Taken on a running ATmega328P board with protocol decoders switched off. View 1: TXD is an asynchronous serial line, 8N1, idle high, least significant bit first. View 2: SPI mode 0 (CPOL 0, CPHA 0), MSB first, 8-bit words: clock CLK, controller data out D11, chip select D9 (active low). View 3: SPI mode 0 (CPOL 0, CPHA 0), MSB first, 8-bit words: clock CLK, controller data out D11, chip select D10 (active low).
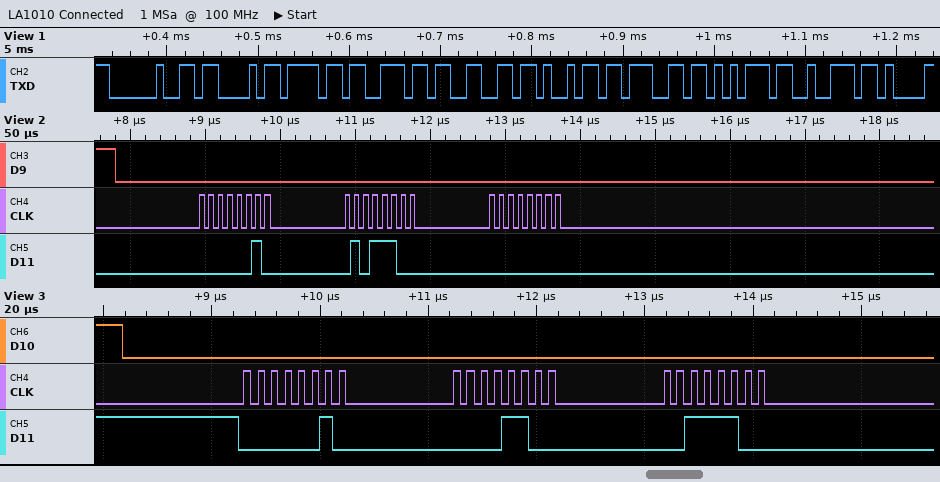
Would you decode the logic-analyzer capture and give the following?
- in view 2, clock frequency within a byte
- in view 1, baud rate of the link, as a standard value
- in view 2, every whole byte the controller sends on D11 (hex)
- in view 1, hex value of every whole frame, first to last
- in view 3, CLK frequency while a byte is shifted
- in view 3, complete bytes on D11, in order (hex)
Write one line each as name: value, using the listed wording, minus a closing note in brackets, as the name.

in view 2, clock frequency within a byte: 8 MHz
in view 1, baud rate of the link, as a standard value: 115200 baud
in view 2, every whole byte the controller sends on D11: 02 5C 00
in view 1, hex value of every whole frame, first to last: 0x20 0x43 0x6F 0x6E 0x66 0x69 0x67 0x75 0x72
in view 3, CLK frequency while a byte is shifted: 8 MHz
in view 3, complete bytes on D11, in order: 0x02 0x0C 0x3C
